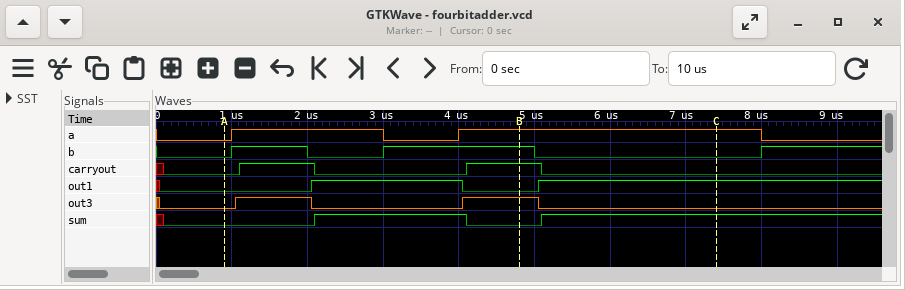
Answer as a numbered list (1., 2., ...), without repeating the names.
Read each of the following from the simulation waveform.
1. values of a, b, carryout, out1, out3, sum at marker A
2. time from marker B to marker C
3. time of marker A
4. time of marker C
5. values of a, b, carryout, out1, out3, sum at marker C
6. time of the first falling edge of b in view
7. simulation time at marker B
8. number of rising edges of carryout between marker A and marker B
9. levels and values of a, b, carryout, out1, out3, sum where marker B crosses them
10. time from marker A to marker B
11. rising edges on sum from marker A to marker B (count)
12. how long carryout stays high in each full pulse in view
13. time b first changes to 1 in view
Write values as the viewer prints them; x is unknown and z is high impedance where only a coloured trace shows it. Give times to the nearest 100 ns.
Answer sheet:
1. a=0, b=0, carryout=0, out1=0, out3=0, sum=0
2. 2600 ns
3. 900 ns
4. 7400 ns
5. a=1, b=0, carryout=0, out1=1, out3=0, sum=1
6. 2000 ns
7. 4800 ns
8. 2
9. a=1, b=1, carryout=1, out1=0, out3=1, sum=0
10. 3900 ns
11. 1
12. 1000 ns, 1000 ns
13. 1000 ns
